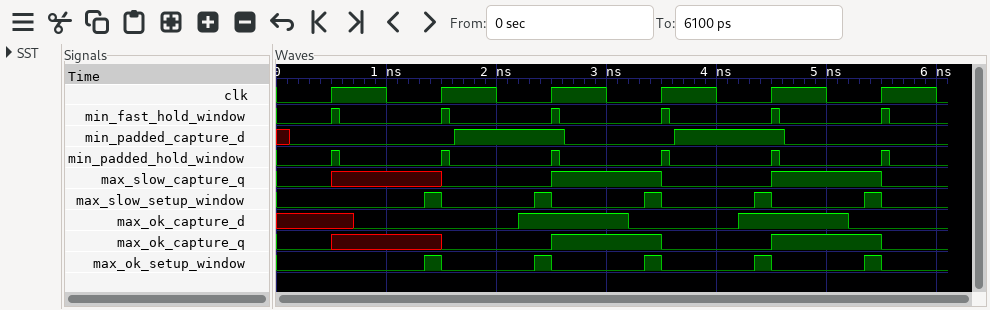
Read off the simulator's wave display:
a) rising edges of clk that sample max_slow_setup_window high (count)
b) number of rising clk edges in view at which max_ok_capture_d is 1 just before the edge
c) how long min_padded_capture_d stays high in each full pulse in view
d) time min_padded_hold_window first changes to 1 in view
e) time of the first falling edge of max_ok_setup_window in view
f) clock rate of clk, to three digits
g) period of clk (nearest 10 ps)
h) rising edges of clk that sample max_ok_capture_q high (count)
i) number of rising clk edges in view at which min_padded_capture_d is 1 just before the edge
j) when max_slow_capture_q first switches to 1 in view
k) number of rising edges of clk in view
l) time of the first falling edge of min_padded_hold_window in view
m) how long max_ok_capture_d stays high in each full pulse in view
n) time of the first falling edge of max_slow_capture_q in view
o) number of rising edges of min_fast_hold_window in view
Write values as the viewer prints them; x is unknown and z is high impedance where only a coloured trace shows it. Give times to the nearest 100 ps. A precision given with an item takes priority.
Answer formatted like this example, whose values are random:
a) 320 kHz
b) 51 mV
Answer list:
a) 5
b) 2
c) 1000 ps, 1000 ps
d) 500 ps
e) 1500 ps
f) 1.00 GHz
g) 1000 ps
h) 2
i) 2
j) 2500 ps
k) 6
l) 600 ps
m) 1000 ps, 1000 ps
n) 3500 ps
o) 6
